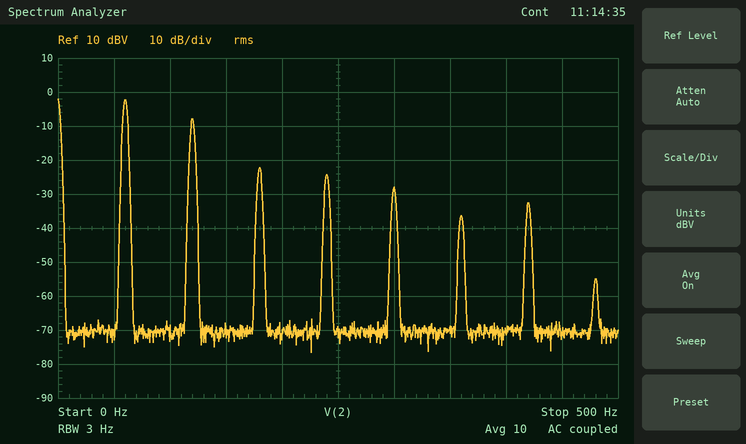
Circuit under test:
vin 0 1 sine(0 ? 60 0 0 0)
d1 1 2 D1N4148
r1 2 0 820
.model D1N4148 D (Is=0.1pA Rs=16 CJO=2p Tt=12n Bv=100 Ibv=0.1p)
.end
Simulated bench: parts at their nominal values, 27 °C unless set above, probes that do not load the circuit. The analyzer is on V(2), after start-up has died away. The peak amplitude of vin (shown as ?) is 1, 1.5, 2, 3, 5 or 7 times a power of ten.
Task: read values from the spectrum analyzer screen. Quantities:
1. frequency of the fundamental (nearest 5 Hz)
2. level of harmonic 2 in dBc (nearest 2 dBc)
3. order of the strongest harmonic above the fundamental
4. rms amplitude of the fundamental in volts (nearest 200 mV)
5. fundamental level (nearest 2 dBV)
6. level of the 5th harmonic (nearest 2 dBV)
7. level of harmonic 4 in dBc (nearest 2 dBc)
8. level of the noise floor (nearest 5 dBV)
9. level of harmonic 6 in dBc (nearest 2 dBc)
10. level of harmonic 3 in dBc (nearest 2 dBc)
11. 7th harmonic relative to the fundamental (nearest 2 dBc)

60 Hz
-6 dBc
2
800 mV
-2 dBV
-28 dBV
-22 dBc
-70 dBV
-34 dBc
-20 dBc
-30 dBc
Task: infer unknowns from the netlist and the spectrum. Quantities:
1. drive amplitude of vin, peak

3 V
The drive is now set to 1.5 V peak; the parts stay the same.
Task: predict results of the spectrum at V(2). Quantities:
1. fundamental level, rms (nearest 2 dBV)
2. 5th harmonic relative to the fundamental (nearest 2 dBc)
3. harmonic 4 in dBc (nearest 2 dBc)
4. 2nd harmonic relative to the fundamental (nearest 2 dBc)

-12 dBV
-22 dBc
-34 dBc
-4 dBc
